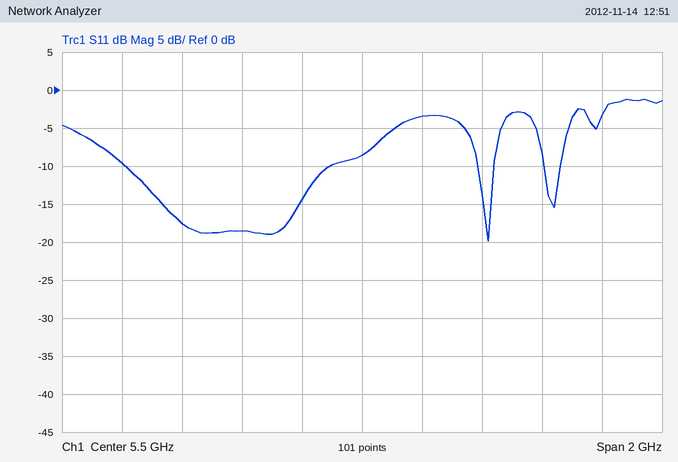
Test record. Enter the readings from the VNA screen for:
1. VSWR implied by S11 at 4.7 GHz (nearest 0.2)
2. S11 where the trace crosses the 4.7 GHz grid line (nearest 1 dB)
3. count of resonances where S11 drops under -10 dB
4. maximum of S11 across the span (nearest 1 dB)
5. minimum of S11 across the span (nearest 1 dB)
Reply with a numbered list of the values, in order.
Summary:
1. 2.0
2. -10 dB
3. 3
4. -1 dB
5. -20 dB
